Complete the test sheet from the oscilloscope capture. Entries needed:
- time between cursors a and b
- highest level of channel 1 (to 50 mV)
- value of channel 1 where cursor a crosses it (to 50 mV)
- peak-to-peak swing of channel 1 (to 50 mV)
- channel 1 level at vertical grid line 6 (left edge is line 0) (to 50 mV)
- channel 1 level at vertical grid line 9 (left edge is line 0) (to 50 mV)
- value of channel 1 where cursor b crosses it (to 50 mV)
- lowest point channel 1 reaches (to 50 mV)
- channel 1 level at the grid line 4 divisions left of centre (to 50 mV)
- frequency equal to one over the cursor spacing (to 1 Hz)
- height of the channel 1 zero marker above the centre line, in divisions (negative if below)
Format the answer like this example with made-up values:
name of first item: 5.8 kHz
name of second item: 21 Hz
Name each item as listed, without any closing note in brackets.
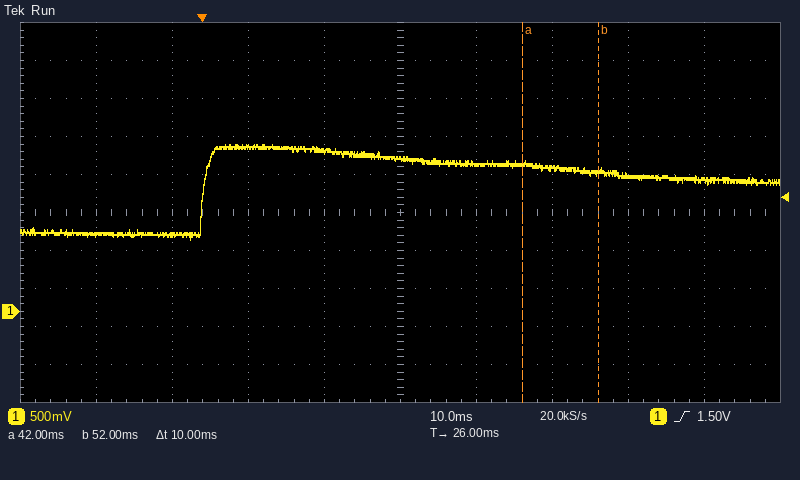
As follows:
time between cursors a and b: 10 ms
highest level of channel 1: 2.20 V
value of channel 1 where cursor a crosses it: 1.95 V
peak-to-peak swing of channel 1: 1.25 V
channel 1 level at vertical grid line 6 (left edge is line 0): 1.95 V
channel 1 level at vertical grid line 9 (left edge is line 0): 1.70 V
value of channel 1 where cursor b crosses it: 1.85 V
lowest point channel 1 reaches: 950 mV
channel 1 level at the grid line 4 divisions left of centre: 1.00 V
frequency equal to one over the cursor spacing: 100 Hz
height of the channel 1 zero marker above the centre line, in divisions: -2.6 div
